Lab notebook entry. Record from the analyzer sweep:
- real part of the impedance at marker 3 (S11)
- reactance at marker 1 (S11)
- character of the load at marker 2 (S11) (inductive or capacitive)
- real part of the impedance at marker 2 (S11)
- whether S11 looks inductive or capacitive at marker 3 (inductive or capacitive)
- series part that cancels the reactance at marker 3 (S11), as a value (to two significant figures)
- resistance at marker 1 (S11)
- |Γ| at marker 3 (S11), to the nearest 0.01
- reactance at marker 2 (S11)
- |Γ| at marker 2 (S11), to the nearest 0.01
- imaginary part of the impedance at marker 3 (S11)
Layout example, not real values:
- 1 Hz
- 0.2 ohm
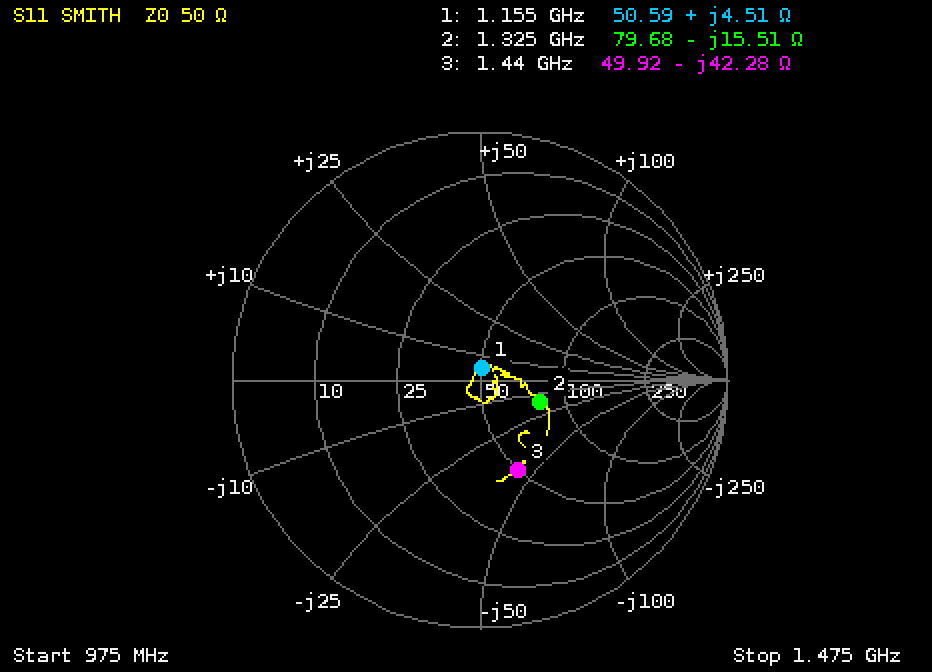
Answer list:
- 49.92 Ω
- +4.51 Ω
- capacitive
- 79.68 Ω
- capacitive
- 4.7 nH
- 50.59 Ω
- 0.39
- -15.51 Ω
- 0.26
- -42.28 Ω
